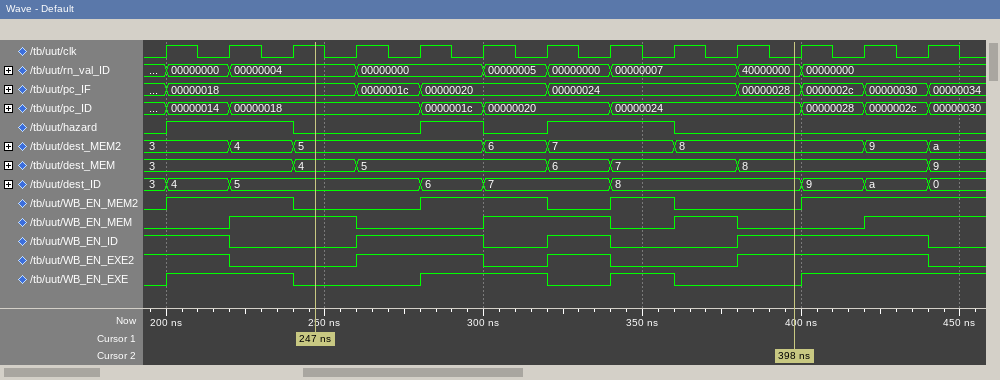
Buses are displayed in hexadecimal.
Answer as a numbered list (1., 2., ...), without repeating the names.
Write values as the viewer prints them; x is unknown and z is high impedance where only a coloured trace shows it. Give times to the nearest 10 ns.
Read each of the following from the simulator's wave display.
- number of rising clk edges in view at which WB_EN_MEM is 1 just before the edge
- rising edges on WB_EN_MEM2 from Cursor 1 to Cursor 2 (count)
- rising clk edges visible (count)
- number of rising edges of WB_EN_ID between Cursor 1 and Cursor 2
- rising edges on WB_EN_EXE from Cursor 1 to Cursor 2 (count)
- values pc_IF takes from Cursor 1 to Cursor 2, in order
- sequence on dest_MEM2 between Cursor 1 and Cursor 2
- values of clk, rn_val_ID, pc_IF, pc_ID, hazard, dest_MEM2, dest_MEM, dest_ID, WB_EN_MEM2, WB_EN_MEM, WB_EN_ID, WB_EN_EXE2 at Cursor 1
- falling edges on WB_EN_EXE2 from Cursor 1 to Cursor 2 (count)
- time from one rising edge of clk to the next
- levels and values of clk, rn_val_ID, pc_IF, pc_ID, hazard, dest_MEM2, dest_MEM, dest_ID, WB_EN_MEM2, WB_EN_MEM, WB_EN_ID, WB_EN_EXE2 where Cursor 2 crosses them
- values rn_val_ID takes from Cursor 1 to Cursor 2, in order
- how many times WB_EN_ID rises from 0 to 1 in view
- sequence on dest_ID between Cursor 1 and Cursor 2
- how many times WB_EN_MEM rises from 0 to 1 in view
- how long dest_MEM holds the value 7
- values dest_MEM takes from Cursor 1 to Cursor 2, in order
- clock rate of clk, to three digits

1. 6
2. 2
3. 13
4. 3
5. 2
6. 00000018, 0000001c, 00000020, 00000024, 00000028
7. 5, 6, 7, 8
8. clk=1, rn_val_ID=00000004, pc_IF=00000018, pc_ID=00000018, hazard=0, dest_MEM2=5, dest_MEM=4, dest_ID=5, WB_EN_MEM2=0, WB_EN_MEM=1, WB_EN_ID=0, WB_EN_EXE2=0
9. 2
10. 20 ns
11. clk=0, rn_val_ID=40000000, pc_IF=00000028, pc_ID=00000024, hazard=0, dest_MEM2=8, dest_MEM=8, dest_ID=8, WB_EN_MEM2=0, WB_EN_MEM=0, WB_EN_ID=1, WB_EN_EXE2=1
12. 00000004, 00000000, 00000005, 00000000, 00000007, 40000000
13. 3
14. 5, 6, 7, 8
15. 4
16. 40 ns
17. 4, 5, 6, 7, 8
18. 50.0 MHz
